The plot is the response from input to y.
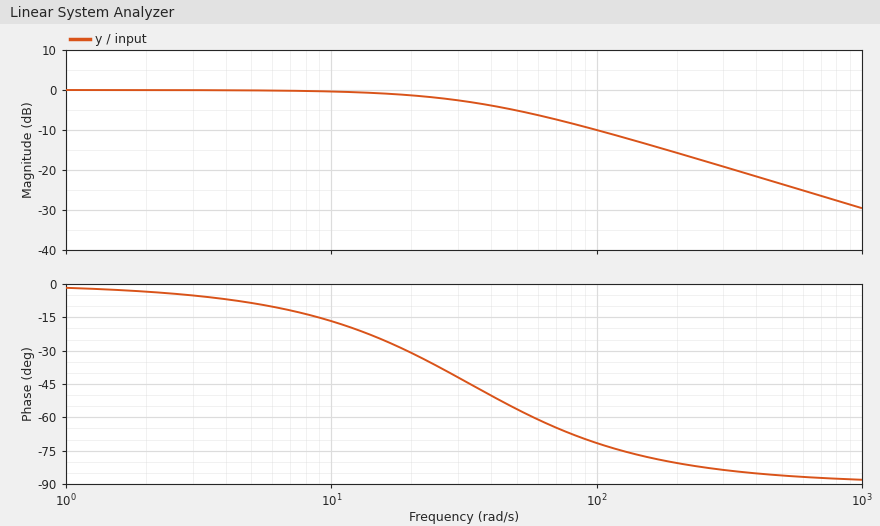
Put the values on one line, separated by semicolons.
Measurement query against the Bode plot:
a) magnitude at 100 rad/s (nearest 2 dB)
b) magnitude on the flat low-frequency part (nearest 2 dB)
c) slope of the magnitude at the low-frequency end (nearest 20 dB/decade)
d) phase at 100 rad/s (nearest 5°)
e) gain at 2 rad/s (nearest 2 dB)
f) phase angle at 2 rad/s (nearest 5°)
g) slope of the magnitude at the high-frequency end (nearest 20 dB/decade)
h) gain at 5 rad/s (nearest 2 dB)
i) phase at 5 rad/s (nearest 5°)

-10 dB; 0 dB; 0 dB/decade; -70°; 0 dB; -5°; -20 dB/decade; 0 dB; -10°
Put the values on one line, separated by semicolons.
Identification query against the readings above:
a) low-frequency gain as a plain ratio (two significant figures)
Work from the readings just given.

1.0
